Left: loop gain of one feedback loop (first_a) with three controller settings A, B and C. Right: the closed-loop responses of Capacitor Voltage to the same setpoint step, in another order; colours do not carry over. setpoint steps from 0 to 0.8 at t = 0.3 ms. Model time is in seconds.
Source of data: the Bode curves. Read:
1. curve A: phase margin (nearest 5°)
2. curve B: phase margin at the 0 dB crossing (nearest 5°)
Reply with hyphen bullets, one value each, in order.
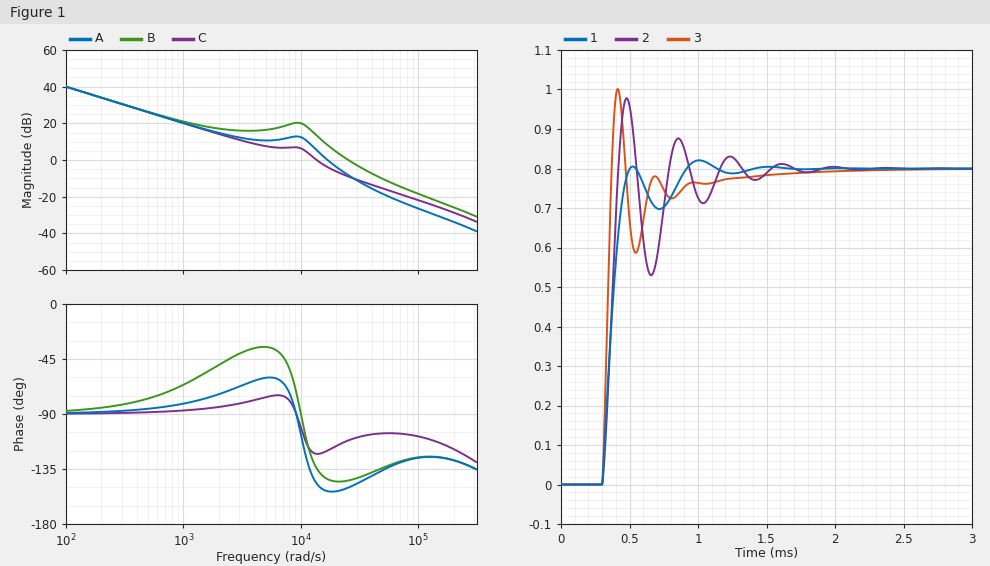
- 25°
- 35°
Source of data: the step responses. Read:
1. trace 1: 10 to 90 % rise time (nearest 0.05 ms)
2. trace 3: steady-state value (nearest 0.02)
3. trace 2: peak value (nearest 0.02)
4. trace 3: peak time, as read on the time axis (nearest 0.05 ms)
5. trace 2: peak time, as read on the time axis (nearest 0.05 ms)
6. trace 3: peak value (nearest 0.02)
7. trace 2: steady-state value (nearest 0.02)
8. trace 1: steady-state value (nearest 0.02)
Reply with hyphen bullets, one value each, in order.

- 0.15 ms
- 0.80
- 0.98
- 0.40 ms
- 0.50 ms
- 1.00
- 0.80
- 0.80
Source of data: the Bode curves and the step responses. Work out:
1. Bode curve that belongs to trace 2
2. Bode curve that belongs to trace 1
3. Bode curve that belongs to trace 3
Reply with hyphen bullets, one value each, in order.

- A
- C
- B
